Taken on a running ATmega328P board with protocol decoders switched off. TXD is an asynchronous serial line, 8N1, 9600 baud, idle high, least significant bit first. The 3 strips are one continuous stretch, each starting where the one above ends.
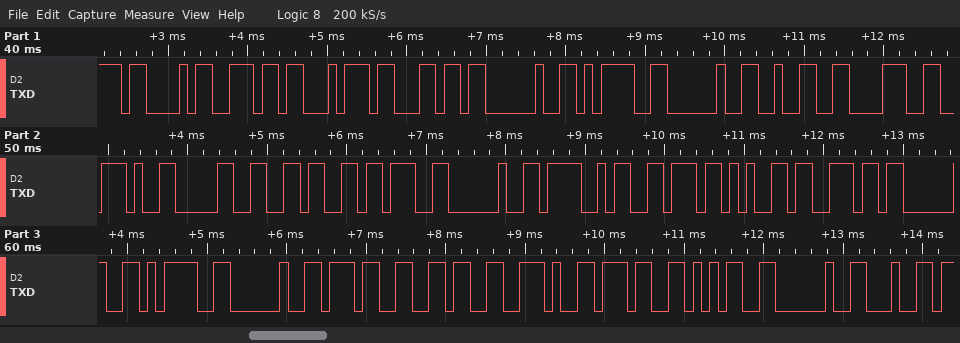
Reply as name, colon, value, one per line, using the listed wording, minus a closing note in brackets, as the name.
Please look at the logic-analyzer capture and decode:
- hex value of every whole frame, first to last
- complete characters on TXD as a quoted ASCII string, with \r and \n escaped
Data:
hex value of every whole frame, first to last: 43 6E 74 6C 20 3D 20 32 38 2E 30 36 3B 20 4F 76 65 6E 20 3D 20 37 36 2E 37 35 20 64
complete characters on TXD as a quoted ASCII string, with \r and \n escaped: "Cntl = 28.06; Oven = 76.75 d"
